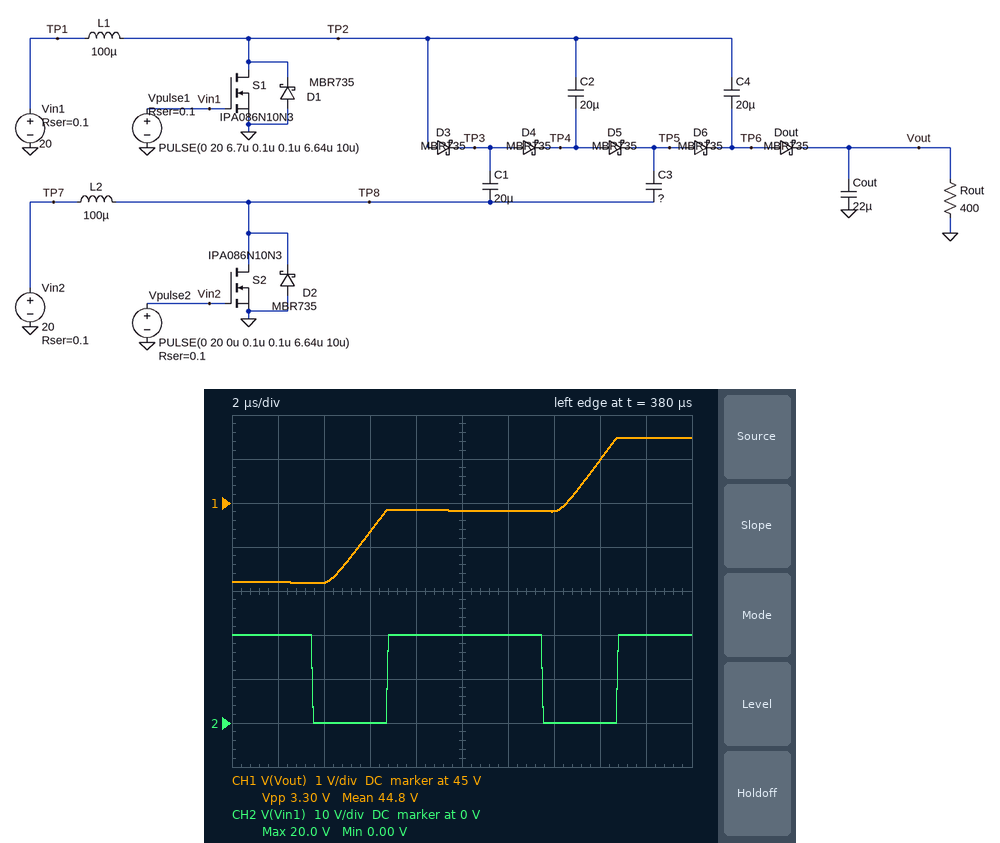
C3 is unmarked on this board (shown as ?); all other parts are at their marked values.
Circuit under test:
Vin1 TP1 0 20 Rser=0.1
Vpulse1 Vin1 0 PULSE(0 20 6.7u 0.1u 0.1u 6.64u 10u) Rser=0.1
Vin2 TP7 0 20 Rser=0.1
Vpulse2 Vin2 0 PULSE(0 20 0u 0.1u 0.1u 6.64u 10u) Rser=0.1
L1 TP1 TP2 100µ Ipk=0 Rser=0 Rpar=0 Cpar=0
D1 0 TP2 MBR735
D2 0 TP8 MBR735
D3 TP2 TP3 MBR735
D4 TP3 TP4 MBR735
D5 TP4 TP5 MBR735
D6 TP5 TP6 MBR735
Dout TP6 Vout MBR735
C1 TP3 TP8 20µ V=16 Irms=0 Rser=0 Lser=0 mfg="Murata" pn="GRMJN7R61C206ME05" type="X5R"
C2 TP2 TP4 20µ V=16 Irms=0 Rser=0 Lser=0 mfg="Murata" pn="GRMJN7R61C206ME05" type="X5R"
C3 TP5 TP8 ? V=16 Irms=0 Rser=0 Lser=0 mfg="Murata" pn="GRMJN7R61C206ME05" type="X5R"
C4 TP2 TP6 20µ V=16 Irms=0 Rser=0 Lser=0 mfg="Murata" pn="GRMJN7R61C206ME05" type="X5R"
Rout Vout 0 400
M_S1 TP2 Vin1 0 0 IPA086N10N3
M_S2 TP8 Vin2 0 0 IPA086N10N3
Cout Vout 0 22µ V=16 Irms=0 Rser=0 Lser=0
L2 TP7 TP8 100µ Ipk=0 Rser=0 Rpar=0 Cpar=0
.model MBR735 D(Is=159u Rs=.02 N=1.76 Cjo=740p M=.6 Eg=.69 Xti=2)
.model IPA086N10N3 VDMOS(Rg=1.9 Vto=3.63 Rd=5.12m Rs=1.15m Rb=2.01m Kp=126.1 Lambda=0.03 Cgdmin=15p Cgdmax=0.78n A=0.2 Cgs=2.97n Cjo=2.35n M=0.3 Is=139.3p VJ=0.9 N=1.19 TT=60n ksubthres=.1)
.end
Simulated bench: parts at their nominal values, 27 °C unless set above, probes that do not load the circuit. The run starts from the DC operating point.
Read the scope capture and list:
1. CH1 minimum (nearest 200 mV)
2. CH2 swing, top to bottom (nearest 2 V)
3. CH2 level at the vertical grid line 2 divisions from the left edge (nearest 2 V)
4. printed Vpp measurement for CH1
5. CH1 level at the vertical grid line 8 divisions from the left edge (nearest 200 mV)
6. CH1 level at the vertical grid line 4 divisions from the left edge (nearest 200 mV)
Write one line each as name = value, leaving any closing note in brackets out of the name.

CH1 minimum = 43.2 V
CH2 swing, top to bottom = 20 V
CH2 level at the vertical grid line 2 divisions from the left edge = 0 V
printed Vpp measurement for CH1 = 3.30 V
CH1 level at the vertical grid line 8 divisions from the left edge = 46.0 V
CH1 level at the vertical grid line 4 divisions from the left edge = 44.8 V
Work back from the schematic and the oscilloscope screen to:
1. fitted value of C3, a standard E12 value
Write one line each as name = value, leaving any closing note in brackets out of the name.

fitted value of C3, a standard E12 value = 27 µF
